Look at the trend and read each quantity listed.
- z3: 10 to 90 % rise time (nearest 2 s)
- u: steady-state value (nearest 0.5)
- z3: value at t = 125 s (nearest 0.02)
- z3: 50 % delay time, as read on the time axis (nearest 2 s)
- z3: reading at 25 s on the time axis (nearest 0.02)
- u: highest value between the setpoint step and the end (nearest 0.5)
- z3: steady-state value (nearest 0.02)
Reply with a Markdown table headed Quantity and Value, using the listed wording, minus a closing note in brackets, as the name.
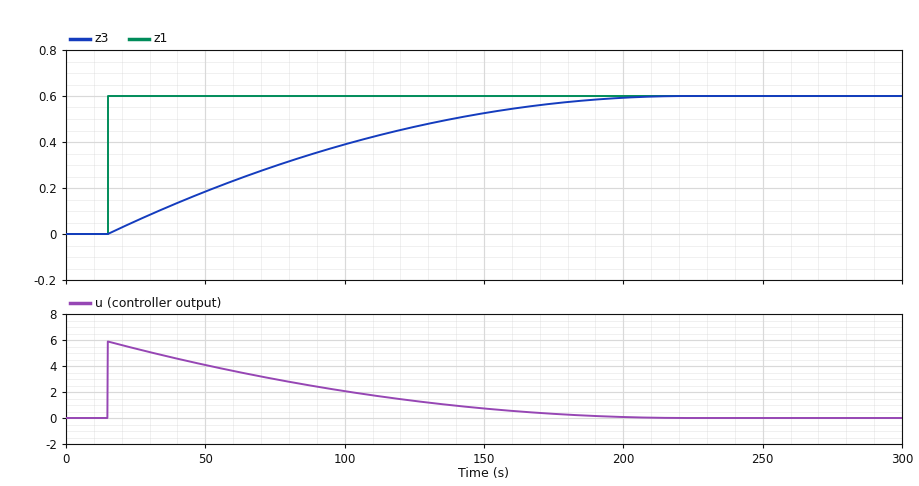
| Quantity | Value |
|---|---|
| z3: 10 to 90 % rise time | 132 s |
| u: steady-state value | 0.0 |
| z3: value at t = 125 s | 0.46 |
| z3: 50 % delay time, as read on the time axis | 76 s |
| z3: reading at 25 s on the time axis | 0.06 |
| u: highest value between the setpoint step and the end | 6.0 |
| z3: steady-state value | 0.60 |
